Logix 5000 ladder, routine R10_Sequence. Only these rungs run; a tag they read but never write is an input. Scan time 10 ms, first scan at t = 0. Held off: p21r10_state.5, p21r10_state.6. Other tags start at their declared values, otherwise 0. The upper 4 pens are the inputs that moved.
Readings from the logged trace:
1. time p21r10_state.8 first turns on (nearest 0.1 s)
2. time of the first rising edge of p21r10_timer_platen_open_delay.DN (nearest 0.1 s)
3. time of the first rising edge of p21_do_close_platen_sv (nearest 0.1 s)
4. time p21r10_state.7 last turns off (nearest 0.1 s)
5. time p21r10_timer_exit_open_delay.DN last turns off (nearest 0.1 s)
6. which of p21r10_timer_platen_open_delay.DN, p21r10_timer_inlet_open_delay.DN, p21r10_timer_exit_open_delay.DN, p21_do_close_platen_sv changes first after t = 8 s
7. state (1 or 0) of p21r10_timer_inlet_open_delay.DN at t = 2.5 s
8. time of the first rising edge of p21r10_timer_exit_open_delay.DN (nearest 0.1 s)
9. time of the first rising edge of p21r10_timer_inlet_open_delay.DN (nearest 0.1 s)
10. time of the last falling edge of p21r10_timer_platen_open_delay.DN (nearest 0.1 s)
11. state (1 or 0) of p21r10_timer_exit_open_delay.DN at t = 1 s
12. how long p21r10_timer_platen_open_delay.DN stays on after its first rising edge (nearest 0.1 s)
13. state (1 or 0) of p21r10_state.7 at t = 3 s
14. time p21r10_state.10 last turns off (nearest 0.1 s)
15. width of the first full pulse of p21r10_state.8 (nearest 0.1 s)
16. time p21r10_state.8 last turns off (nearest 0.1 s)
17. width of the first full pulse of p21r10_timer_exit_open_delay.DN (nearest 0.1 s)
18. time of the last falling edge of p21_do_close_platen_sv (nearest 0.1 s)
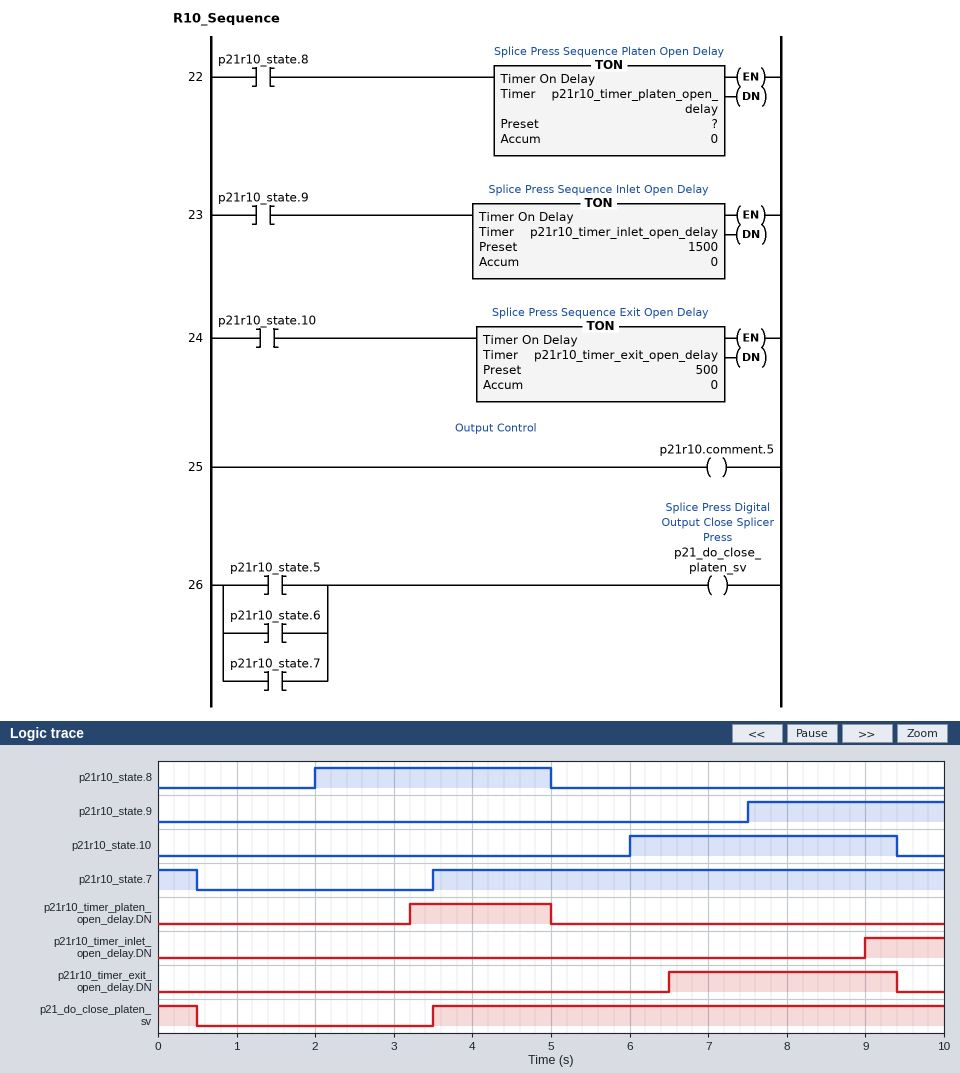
2.0 s
3.2 s
3.5 s
0.5 s
9.4 s
p21r10_timer_inlet_open_delay.DN
0
6.5 s
9.0 s
5.0 s
0
1.8 s
0
9.4 s
3.0 s
5.0 s
2.9 s
0.5 s
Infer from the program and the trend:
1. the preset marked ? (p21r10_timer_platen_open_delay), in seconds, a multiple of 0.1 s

1.2 s
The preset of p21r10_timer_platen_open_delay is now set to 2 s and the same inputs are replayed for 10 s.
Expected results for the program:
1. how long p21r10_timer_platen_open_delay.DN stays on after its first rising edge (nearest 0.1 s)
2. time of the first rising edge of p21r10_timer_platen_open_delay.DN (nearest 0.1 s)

1.0 s
4.0 s
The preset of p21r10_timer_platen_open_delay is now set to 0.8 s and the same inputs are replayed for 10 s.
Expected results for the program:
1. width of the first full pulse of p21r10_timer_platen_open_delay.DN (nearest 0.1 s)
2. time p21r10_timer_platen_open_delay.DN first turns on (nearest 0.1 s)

2.2 s
2.8 s
